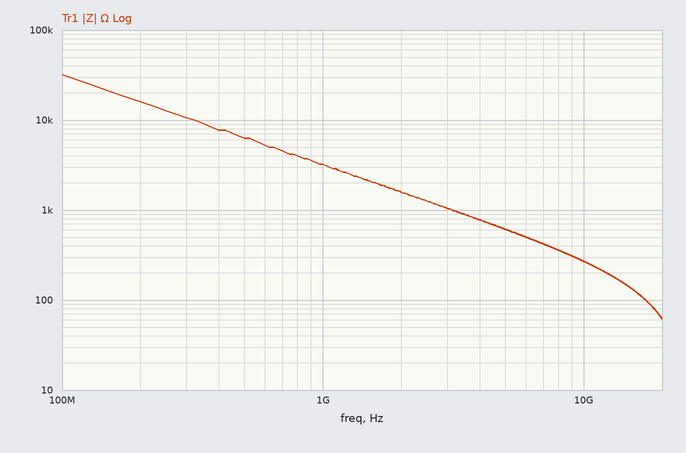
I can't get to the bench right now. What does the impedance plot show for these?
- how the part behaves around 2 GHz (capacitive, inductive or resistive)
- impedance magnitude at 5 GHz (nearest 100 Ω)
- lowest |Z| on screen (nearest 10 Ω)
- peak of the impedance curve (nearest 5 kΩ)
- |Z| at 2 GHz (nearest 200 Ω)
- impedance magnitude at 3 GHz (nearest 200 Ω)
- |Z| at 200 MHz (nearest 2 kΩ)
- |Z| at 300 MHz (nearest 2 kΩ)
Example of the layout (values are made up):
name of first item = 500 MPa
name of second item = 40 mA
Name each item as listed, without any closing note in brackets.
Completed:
how the part behaves around 2 GHz = capacitive
impedance magnitude at 5 GHz = 600 Ω
lowest |Z| on screen = 60 Ω
peak of the impedance curve = 30 kΩ
|Z| at 2 GHz = 1.6 kΩ
impedance magnitude at 3 GHz = 1.0 kΩ
|Z| at 200 MHz = 16 kΩ
|Z| at 300 MHz = 10 kΩ
